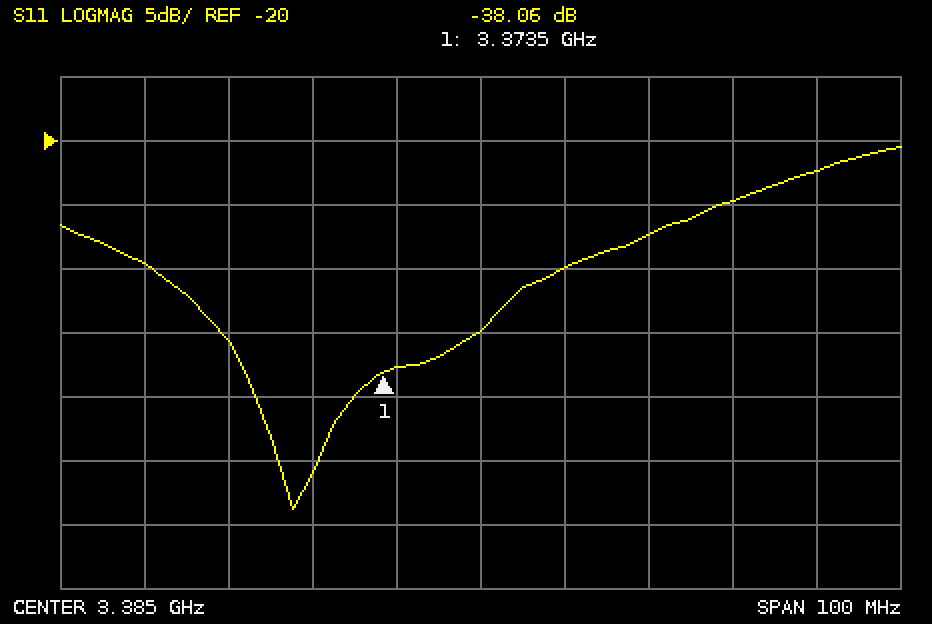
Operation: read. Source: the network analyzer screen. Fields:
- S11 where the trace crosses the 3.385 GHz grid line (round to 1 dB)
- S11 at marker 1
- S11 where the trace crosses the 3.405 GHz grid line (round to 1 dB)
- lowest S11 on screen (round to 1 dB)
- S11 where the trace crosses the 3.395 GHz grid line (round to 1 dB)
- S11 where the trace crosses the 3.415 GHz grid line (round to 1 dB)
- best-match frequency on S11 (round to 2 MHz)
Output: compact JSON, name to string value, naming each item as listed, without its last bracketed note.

{"S11 where the trace crosses the 3.385 GHz grid line": "-35 dB", "S11 at marker 1": "-38.06 dB", "S11 where the trace crosses the 3.405 GHz grid line": "-27 dB", "lowest S11 on screen": "-49 dB", "S11 where the trace crosses the 3.395 GHz grid line": "-30 dB", "S11 where the trace crosses the 3.415 GHz grid line": "-25 dB", "best-match frequency on S11": "3.362 GHz"}
